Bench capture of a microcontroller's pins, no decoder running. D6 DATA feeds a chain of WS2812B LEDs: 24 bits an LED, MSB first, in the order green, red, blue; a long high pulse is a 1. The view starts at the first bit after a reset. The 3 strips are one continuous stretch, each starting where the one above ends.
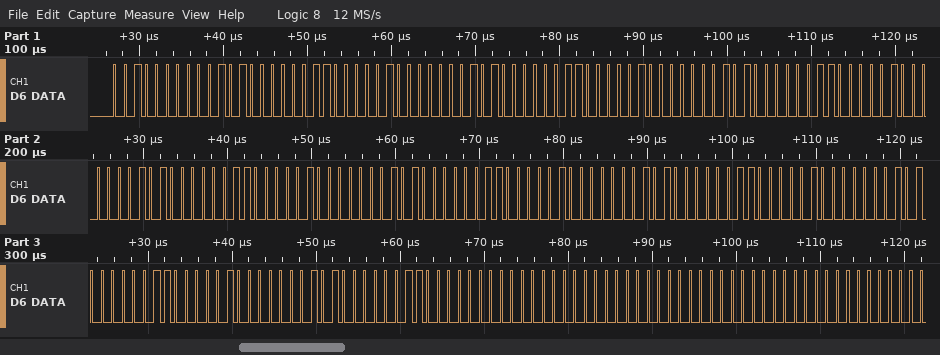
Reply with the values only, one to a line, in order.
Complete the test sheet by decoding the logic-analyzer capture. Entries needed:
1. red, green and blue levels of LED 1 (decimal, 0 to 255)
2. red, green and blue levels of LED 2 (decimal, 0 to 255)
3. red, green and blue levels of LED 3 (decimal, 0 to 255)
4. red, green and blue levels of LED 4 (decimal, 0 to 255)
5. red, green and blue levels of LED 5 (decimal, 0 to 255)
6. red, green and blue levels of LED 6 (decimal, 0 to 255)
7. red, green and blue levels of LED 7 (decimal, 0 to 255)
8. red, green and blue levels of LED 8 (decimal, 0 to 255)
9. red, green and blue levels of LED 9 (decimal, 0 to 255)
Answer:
40, 32, 24
40, 32, 24
40, 32, 24
40, 32, 24
40, 32, 24
40, 32, 24
40, 32, 24
40, 32, 24
0, 0, 0
